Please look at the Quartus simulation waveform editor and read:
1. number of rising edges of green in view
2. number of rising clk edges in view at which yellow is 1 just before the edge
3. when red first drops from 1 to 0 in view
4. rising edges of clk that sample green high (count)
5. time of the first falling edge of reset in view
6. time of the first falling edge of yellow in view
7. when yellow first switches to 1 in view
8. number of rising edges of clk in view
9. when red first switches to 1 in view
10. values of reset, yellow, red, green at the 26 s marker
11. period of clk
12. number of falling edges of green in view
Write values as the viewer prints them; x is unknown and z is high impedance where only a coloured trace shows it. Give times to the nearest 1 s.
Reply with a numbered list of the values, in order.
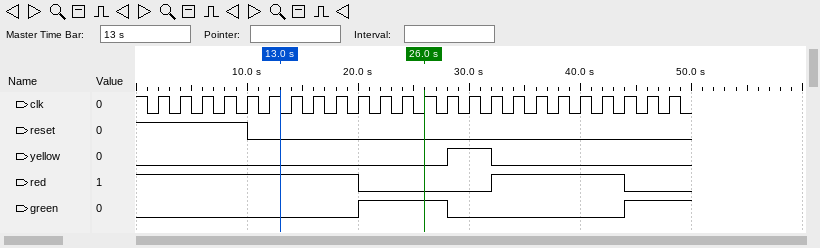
1. 2
2. 2
3. 20 s
4. 6
5. 10 s
6. 32 s
7. 28 s
8. 24
9. 32 s
10. reset=0, yellow=0, red=0, green=1
11. 2 s
12. 1
